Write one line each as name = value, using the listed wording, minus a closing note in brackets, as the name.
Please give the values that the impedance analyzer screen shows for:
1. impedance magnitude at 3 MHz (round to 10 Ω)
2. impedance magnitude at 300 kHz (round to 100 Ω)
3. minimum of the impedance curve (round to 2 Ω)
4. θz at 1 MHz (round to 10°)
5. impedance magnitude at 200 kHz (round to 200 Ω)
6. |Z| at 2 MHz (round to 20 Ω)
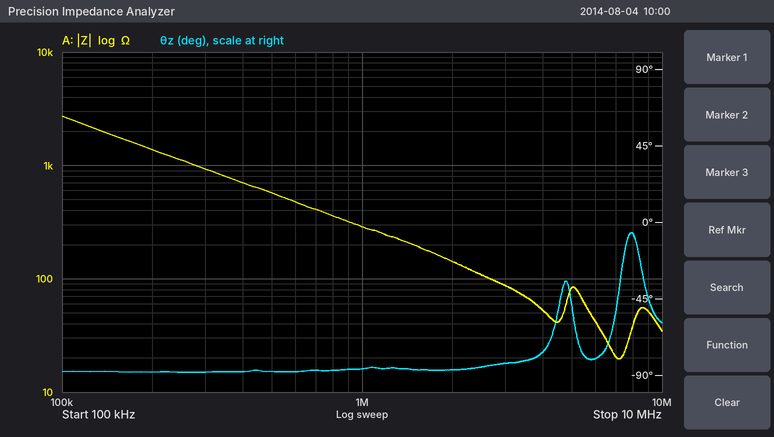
impedance magnitude at 3 MHz = 90 Ω
impedance magnitude at 300 kHz = 900 Ω
minimum of the impedance curve = 20 Ω
θz at 1 MHz = -90°
impedance magnitude at 200 kHz = 1.4 kΩ
|Z| at 2 MHz = 140 Ω
